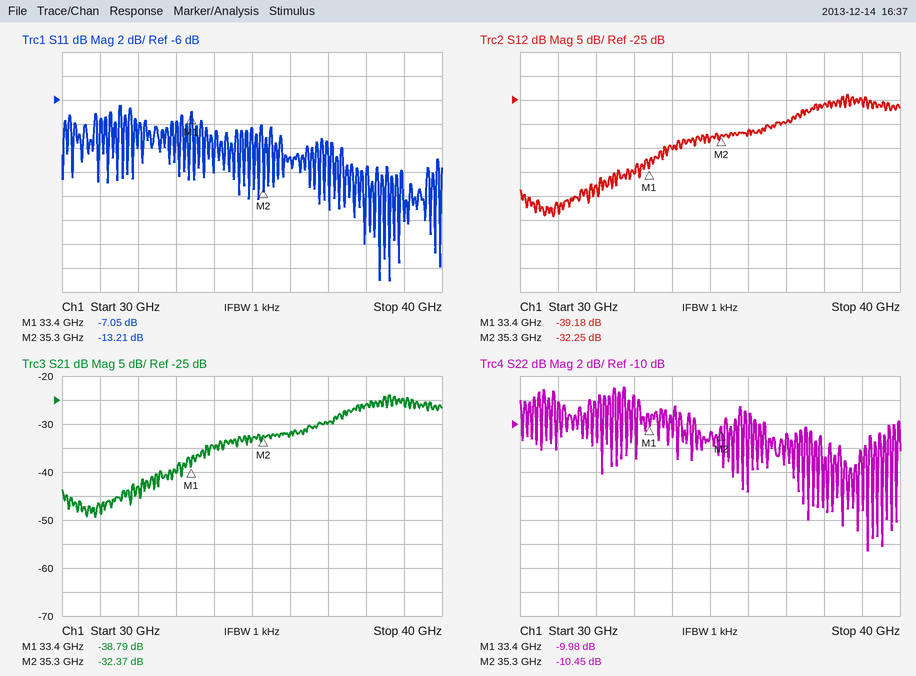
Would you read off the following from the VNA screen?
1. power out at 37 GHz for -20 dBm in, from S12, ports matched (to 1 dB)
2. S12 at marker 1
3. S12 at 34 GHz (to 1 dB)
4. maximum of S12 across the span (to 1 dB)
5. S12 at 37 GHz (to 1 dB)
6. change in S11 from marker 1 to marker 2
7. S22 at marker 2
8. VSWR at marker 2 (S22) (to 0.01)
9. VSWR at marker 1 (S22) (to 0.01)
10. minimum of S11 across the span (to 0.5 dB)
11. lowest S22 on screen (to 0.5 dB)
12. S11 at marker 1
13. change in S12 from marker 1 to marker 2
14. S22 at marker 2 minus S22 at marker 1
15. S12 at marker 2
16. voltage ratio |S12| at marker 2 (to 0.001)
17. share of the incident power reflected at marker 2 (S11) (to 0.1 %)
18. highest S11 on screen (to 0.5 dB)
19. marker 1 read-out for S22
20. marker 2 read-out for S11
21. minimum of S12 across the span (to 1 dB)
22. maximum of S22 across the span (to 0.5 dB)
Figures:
-50 dBm
-39.18 dB
-35 dB
-24 dB
-30 dB
-6.16 dB
-10.45 dB
1.86
1.93
-21.0 dB
-20.5 dB
-7.05 dB
6.93 dB
-0.47 dB
-32.25 dB
0.024
4.8 %
-6.5 dB
-9.98 dB
-13.21 dB
-49 dB
-7.0 dB
